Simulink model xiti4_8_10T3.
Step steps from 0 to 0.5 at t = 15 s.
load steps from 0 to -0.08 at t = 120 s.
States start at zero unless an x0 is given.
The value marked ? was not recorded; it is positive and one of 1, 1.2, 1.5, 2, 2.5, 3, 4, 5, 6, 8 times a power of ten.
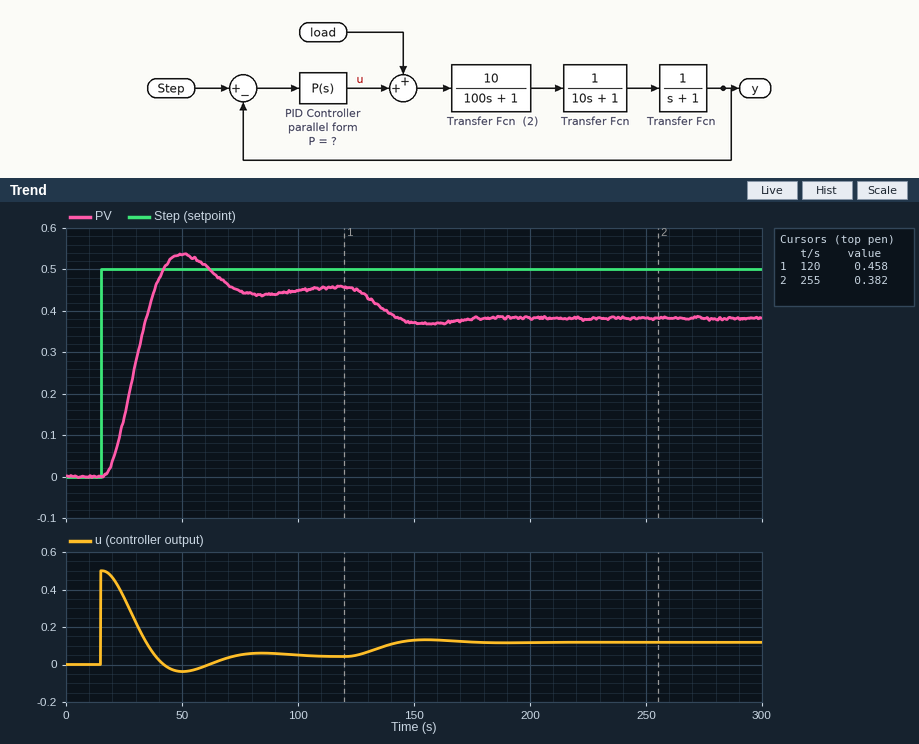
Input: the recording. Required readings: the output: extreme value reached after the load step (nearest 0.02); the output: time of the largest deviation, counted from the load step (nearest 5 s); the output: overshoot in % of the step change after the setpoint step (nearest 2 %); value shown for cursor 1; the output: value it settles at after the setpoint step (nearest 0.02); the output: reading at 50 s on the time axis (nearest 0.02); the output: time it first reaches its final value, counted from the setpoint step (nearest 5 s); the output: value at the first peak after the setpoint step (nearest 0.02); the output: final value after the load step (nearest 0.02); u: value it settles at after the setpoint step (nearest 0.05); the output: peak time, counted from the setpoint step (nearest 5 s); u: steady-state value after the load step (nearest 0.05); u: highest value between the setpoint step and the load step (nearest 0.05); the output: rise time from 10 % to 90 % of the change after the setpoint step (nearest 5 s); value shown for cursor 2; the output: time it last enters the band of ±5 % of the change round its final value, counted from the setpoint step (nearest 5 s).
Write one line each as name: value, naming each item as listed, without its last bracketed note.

the output: extreme value reached after the load step: 0.36
the output: time of the largest deviation, counted from the load step: 35 s
the output: overshoot in % of the step change after the setpoint step: 18 %
value shown for cursor 1: 0.458
the output: value it settles at after the setpoint step: 0.46
the output: reading at 50 s on the time axis: 0.54
the output: time it first reaches its final value, counted from the setpoint step: 25 s
the output: value at the first peak after the setpoint step: 0.54
the output: final value after the load step: 0.38
u: value it settles at after the setpoint step: 0.05
the output: peak time, counted from the setpoint step: 35 s
u: steady-state value after the load step: 0.10
u: highest value between the setpoint step and the load step: 0.50
the output: rise time from 10 % to 90 % of the change after the setpoint step: 15 s
value shown for cursor 2: 0.382
the output: time it last enters the band of ±5 % of the change round its final value, counted from the setpoint step: 50 s
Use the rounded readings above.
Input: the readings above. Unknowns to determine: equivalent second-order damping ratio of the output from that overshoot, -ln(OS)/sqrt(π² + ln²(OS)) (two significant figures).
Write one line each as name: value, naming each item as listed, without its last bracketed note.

equivalent second-order damping ratio of the output from that overshoot, -ln(OS)/sqrt(π² + ln²(OS)): 0.48
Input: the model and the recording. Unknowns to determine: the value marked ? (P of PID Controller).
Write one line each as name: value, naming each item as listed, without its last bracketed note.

the value marked ?: 1
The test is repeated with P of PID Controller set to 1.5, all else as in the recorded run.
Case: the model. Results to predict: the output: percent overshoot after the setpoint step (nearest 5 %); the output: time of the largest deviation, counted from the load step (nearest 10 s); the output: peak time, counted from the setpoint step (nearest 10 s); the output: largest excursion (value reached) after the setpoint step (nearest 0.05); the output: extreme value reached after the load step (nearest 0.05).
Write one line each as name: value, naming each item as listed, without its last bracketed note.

the output: percent overshoot after the setpoint step: 30 %
the output: time of the largest deviation, counted from the load step: 30 s
the output: peak time, counted from the setpoint step: 30 s
the output: largest excursion (value reached) after the setpoint step: 0.60
the output: extreme value reached after the load step: 0.40
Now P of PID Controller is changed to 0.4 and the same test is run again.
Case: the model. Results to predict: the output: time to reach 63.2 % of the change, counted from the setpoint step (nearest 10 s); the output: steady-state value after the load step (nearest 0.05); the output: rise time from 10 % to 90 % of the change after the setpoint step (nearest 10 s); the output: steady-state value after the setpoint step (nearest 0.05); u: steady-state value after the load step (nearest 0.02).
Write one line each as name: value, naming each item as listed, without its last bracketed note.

the output: time to reach 63.2 % of the change, counted from the setpoint step: 30 s
the output: steady-state value after the load step: 0.25
the output: rise time from 10 % to 90 % of the change after the setpoint step: 30 s
the output: steady-state value after the setpoint step: 0.40
u: steady-state value after the load step: 0.10
